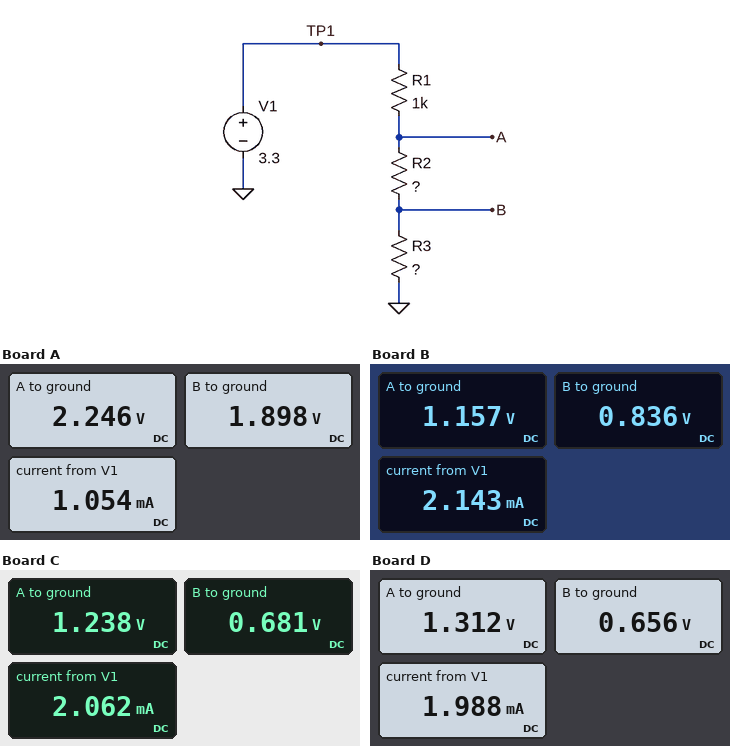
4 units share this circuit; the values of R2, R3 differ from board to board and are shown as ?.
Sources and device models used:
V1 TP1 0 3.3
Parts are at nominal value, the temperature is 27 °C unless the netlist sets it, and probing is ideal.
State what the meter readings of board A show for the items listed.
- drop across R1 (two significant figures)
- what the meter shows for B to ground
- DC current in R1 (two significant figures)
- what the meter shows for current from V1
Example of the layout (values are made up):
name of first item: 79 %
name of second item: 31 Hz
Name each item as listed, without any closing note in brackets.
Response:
drop across R1: 1.1 V
what the meter shows for B to ground: 1.898 V
DC current in R1: 1.1 mA
what the meter shows for current from V1: 1.054 mA
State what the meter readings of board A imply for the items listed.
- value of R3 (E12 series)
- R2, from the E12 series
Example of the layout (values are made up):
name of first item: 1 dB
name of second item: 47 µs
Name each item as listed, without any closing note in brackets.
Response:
value of R3: 1.8 kΩ
R2, from the E12 series: 330 Ω
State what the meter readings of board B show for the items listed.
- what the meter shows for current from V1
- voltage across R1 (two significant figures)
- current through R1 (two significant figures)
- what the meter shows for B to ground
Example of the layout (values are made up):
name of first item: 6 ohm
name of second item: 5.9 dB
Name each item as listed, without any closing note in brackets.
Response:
what the meter shows for current from V1: 2.143 mA
voltage across R1: 2.1 V
current through R1: 2.1 mA
what the meter shows for B to ground: 0.836 V
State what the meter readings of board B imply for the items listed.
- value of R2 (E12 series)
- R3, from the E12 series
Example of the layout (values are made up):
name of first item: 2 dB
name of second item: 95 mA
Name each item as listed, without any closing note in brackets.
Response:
value of R2: 150 Ω
R3, from the E12 series: 390 Ω
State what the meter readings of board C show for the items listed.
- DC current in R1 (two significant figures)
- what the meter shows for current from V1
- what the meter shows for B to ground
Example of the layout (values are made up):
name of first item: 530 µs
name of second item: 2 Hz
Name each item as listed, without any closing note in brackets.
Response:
DC current in R1: 2.1 mA
what the meter shows for current from V1: 2.062 mA
what the meter shows for B to ground: 0.681 V
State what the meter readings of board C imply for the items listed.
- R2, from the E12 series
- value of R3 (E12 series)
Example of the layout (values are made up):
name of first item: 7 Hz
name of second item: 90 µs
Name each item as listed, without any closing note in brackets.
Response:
R2, from the E12 series: 270 Ω
value of R3: 330 Ω
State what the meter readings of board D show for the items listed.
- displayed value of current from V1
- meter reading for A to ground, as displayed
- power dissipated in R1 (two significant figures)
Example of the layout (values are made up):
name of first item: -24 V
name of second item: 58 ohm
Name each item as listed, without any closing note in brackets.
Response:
displayed value of current from V1: 1.988 mA
meter reading for A to ground, as displayed: 1.312 V
power dissipated in R1: 4.0 mW
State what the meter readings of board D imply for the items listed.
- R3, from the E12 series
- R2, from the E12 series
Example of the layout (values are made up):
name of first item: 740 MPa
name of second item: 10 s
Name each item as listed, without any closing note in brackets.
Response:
R3, from the E12 series: 330 Ω
R2, from the E12 series: 330 Ω
